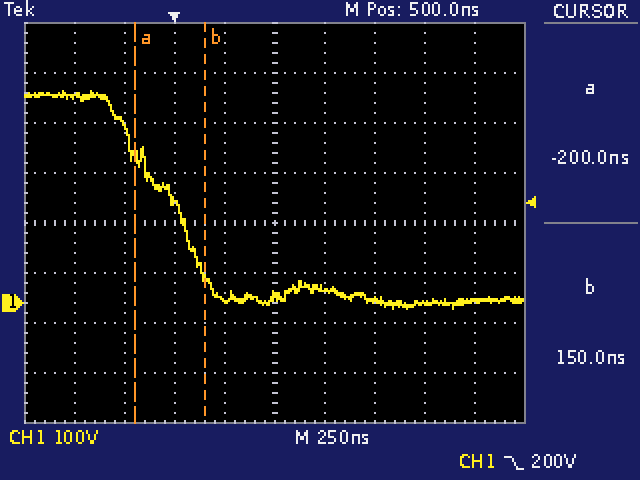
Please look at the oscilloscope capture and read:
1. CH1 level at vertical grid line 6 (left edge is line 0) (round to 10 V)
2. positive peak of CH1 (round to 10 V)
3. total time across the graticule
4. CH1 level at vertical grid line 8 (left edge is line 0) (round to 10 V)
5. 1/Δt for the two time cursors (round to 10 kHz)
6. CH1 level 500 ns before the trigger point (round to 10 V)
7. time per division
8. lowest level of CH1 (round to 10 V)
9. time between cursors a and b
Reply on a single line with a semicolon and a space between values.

30 V; 420 V; 2.5 µs; 0 V; 2.86 MHz; 410 V; 250 ns; -10 V; 350 ns
